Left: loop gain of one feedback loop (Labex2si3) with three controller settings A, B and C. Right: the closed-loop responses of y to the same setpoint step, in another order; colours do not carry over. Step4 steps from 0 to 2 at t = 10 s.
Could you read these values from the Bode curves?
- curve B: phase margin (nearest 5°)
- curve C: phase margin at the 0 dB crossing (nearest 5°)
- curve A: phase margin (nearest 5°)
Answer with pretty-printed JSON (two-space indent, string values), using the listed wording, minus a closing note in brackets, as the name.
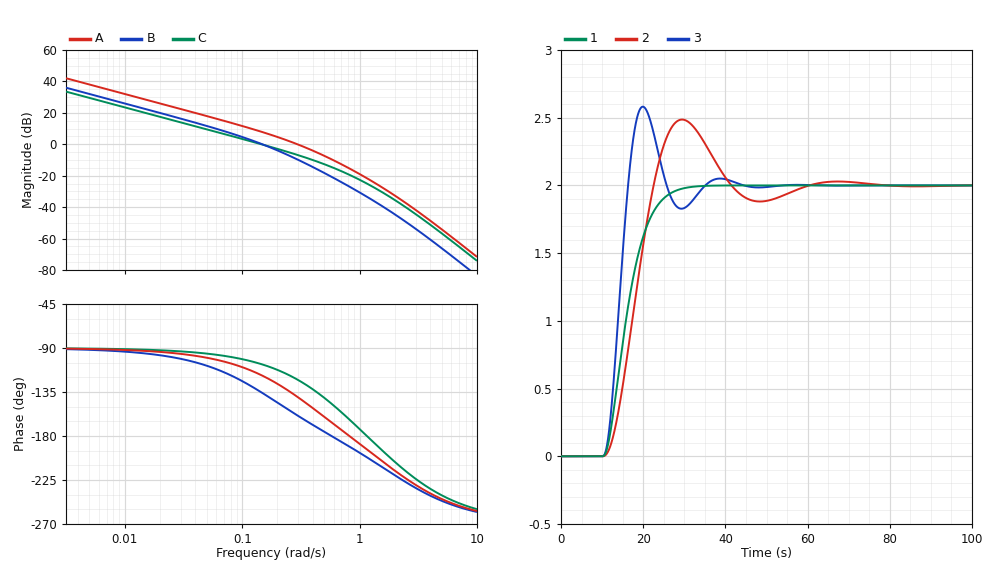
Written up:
{
  "curve B: phase margin": "45°",
  "curve C: phase margin at the 0 dB crossing": "75°",
  "curve A: phase margin": "40°"
}
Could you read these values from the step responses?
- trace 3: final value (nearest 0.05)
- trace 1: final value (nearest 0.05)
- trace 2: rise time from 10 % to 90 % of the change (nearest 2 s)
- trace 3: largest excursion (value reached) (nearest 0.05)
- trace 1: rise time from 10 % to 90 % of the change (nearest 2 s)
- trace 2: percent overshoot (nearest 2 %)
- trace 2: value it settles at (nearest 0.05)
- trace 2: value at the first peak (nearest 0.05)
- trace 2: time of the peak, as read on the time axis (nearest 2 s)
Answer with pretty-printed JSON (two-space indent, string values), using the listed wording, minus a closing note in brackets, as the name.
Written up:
{
  "trace 3: final value": "2.00",
  "trace 1: final value": "2.00",
  "trace 2: rise time from 10 % to 90 % of the change": "8 s",
  "trace 3: largest excursion (value reached)": "2.60",
  "trace 1: rise time from 10 % to 90 % of the change": "10 s",
  "trace 2: percent overshoot": "24 %",
  "trace 2: value it settles at": "2.00",
  "trace 2: value at the first peak": "2.50",
  "trace 2: time of the peak, as read on the time axis": "30 s"
}
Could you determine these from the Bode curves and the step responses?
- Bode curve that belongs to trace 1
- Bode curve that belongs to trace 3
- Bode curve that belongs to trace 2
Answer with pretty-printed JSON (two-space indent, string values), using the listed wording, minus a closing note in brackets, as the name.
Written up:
{
  "Bode curve that belongs to trace 1": "C",
  "Bode curve that belongs to trace 3": "A",
  "Bode curve that belongs to trace 2": "B"
}
